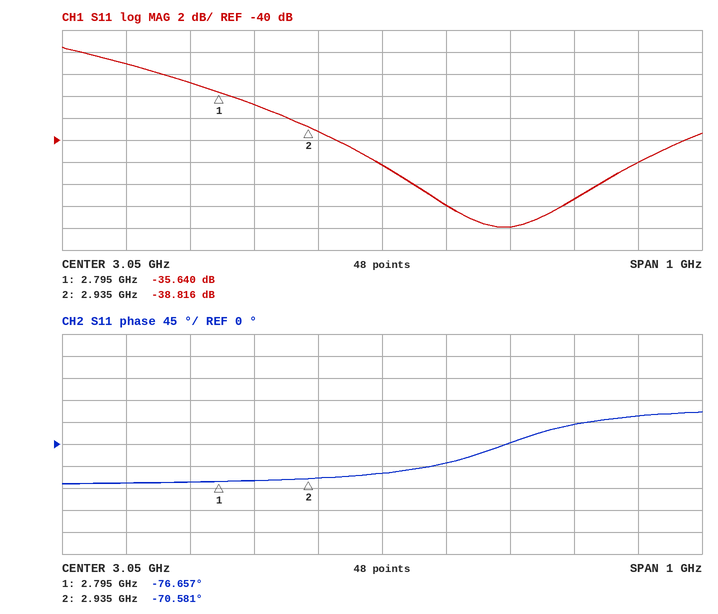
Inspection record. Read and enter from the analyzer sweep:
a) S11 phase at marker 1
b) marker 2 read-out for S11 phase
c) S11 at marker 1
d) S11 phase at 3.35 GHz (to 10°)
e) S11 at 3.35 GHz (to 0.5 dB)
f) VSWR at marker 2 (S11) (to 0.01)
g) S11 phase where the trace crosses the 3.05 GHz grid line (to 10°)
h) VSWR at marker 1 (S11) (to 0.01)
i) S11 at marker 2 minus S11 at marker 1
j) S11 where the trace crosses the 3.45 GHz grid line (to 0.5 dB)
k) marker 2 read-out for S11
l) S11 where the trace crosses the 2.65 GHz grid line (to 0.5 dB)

-76.657°
-70.581°
-35.640 dB
40°
-45.5 dB
1.02
-60°
1.03
-3.176 dB
-42.0 dB
-38.816 dB
-33.0 dB
